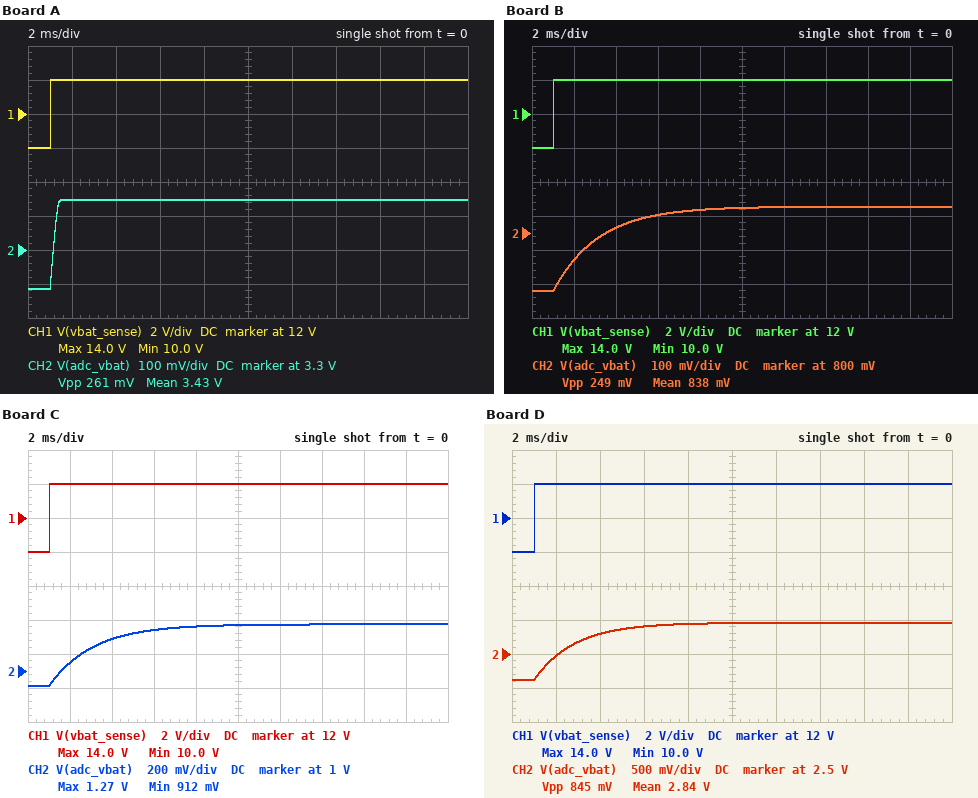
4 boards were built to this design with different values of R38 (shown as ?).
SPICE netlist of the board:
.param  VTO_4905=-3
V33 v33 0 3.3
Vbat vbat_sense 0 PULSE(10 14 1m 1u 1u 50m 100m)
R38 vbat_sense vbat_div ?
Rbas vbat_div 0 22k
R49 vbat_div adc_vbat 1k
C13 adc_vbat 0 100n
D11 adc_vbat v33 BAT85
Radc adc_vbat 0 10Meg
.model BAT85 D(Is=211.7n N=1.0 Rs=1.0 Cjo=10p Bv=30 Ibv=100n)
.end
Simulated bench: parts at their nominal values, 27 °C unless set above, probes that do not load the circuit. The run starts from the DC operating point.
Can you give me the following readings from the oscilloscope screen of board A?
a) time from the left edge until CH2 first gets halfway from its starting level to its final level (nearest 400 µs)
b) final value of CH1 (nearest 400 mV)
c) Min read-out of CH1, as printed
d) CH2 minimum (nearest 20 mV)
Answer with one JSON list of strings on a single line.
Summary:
["1.2 ms", "14.0 V", "10.0 V", "3.18 V"]
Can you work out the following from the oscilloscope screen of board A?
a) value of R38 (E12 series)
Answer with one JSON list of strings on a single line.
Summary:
["47 kΩ"]
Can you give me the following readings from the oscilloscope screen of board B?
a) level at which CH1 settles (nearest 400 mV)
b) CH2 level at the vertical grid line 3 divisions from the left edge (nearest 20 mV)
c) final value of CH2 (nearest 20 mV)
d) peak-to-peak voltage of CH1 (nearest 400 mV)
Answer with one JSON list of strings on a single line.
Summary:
["14.0 V", "860 mV", "880 mV", "4.0 V"]
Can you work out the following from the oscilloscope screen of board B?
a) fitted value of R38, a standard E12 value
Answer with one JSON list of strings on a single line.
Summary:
["330 kΩ"]
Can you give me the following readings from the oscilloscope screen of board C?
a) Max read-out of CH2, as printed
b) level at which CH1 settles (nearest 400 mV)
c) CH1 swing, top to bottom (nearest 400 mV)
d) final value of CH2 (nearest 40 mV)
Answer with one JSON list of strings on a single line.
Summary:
["1.27 V", "14.0 V", "4.0 V", "1.28 V"]
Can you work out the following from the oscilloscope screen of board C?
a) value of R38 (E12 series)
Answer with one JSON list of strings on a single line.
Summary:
["220 kΩ"]
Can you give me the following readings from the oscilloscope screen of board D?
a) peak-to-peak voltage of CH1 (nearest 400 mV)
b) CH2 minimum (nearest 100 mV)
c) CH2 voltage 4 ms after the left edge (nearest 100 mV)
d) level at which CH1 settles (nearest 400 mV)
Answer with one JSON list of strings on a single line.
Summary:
["4.0 V", "2.1 V", "2.8 V", "14.0 V"]
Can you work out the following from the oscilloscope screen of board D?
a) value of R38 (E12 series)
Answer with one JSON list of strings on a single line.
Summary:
["82 kΩ"]
